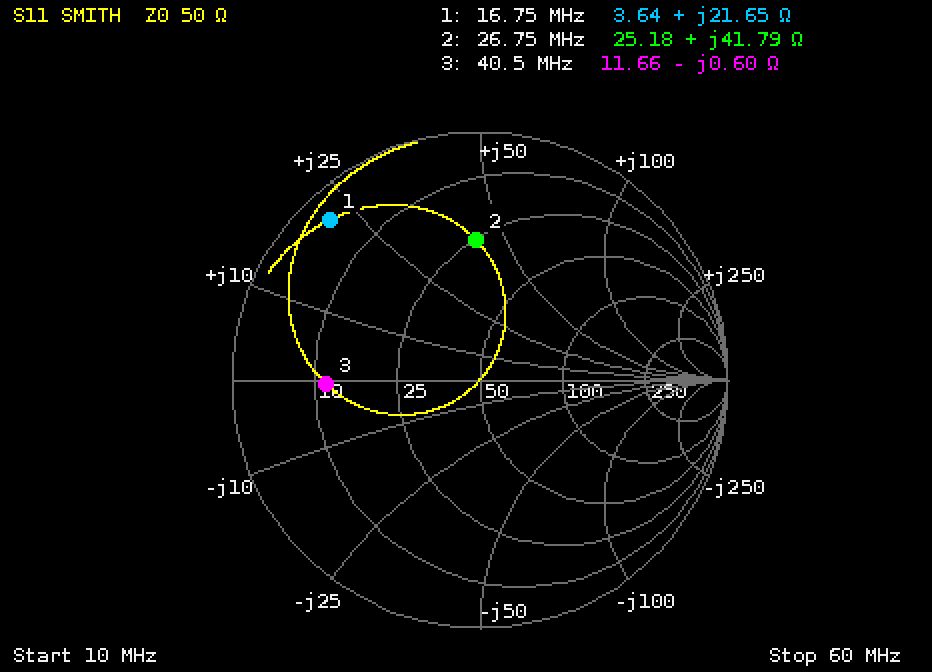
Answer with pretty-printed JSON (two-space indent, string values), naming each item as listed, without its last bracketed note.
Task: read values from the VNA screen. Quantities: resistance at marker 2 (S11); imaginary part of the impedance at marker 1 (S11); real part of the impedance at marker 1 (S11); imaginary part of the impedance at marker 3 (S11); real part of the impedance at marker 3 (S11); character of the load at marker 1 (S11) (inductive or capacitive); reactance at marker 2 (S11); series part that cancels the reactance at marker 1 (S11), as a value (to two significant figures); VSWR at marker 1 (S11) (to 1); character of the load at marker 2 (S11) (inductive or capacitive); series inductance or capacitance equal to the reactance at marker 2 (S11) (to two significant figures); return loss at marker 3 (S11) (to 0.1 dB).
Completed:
{
  "resistance at marker 2": "25.18 Ω",
  "imaginary part of the impedance at marker 1": "+21.65 Ω",
  "real part of the impedance at marker 1": "3.64 Ω",
  "imaginary part of the impedance at marker 3": "-0.60 Ω",
  "real part of the impedance at marker 3": "11.66 Ω",
  "character of the load at marker 1 (S11)": "inductive",
  "reactance at marker 2": "+41.79 Ω",
  "series part that cancels the reactance at marker 1 (S11), as a value": "440 pF",
  "VSWR at marker 1 (S11)": "16",
  "character of the load at marker 2 (S11)": "inductive",
  "series inductance or capacitance equal to the reactance at marker 2 (S11)": "250 nH",
  "return loss at marker 3 (S11)": "4.1 dB"
}
